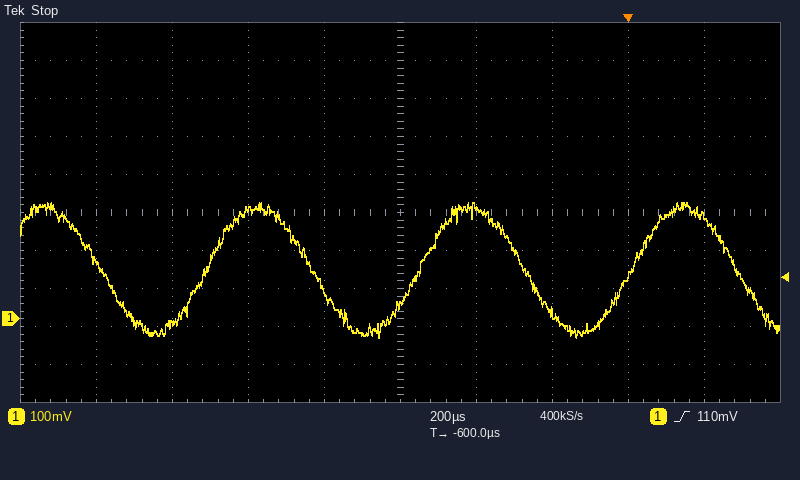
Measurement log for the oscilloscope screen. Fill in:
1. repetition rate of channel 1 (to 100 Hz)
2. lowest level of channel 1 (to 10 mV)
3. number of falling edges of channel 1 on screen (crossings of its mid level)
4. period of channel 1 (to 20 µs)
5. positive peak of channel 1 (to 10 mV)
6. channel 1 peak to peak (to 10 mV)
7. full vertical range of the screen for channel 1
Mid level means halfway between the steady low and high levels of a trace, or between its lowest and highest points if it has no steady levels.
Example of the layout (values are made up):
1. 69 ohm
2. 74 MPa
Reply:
1. 1.8 kHz
2. -50 mV
3. 4
4. 560 µs
5. 310 mV
6. 360 mV
7. 1 V
